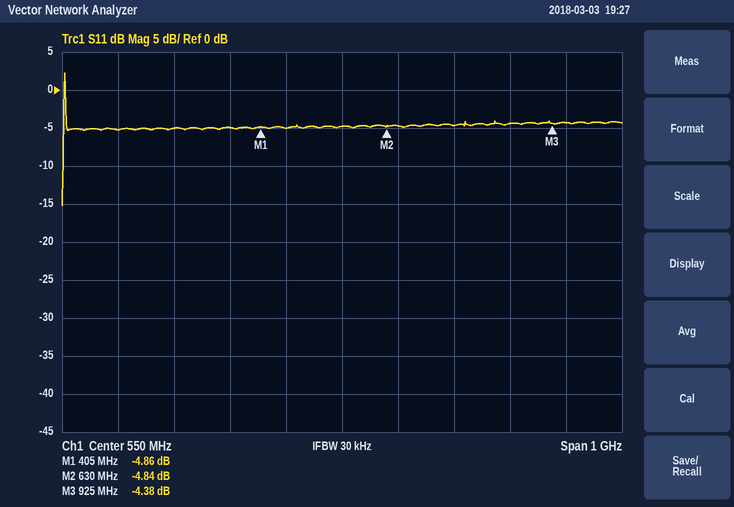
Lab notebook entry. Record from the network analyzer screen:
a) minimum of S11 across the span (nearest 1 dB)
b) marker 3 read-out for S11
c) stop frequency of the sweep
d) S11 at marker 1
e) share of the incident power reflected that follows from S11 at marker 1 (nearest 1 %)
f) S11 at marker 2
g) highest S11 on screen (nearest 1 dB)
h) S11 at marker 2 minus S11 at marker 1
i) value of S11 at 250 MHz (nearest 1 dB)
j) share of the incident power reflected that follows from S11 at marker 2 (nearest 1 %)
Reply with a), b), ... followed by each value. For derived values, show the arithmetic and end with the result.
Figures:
a) -15 dB
b) -4.38 dB
c) 1.05 GHz
d) -4.86 dB
e) 10^(-4.86/10) ≈ 33 %
f) -4.84 dB
g) 2 dB
h) -4.84 − (-4.86) = 0.02 dB
i) -5 dB
j) 10^(-4.84/10) ≈ 33 %
